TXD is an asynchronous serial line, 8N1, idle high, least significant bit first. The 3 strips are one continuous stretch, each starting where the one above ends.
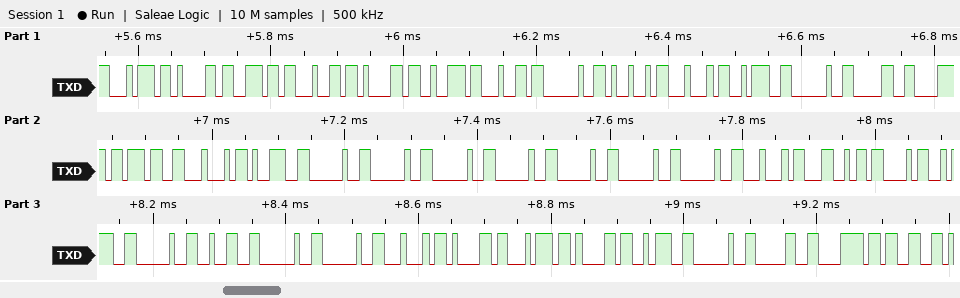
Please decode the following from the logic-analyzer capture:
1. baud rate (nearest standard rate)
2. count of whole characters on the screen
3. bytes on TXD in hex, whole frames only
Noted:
115200 baud
41
0x74 0x61 0x6E 0x64 0x61 0x72 0x64 0x20 0x49 0x44 0x3A 0x20 0x30 0x78 0x37 0x44 0x39 0x20 0x20 0x20 0x20 0x20 0x20 0x20 0x44 0x4C 0x43 0x3A 0x20 0x32 0x20 0x20 0x44 0x61 0x74 0x61 0x3A 0x20 0x30 0x78 0x33
